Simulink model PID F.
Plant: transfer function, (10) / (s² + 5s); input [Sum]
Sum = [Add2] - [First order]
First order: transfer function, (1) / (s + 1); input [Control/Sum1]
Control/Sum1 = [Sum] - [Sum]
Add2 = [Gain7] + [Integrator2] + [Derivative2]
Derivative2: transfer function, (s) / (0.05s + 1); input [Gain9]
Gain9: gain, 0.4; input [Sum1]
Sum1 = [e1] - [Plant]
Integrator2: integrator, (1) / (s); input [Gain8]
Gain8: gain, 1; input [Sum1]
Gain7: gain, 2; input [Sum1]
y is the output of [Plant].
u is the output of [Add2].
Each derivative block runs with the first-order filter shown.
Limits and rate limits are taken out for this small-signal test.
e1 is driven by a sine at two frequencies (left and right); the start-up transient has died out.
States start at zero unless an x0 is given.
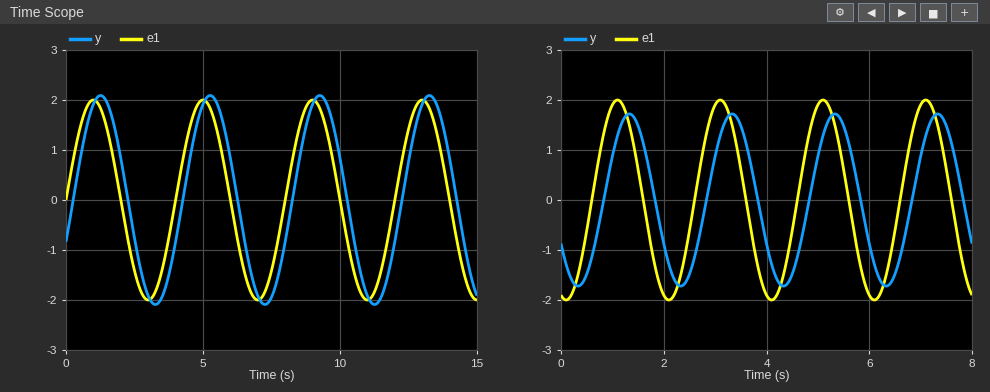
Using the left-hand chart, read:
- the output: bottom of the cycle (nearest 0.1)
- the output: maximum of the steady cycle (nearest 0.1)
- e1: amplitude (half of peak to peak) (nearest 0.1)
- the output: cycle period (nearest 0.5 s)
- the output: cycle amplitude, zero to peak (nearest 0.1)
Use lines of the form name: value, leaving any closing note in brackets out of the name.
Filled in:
the output: bottom of the cycle: -2.1
the output: maximum of the steady cycle: 2.1
e1: amplitude (half of peak to peak): 2.0
the output: cycle period: 4.0 s
the output: cycle amplitude, zero to peak: 2.1
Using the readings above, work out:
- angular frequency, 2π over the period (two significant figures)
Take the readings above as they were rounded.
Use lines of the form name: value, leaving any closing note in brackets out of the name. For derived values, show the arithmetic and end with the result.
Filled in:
angular frequency, 2π over the period: 2π / 4 = 1.6 rad/s
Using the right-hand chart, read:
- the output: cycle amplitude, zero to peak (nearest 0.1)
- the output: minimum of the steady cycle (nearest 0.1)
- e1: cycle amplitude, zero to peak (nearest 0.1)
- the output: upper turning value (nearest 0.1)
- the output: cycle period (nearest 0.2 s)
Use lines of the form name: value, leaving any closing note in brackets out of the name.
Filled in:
the output: cycle amplitude, zero to peak: 1.7
the output: minimum of the steady cycle: -1.7
e1: cycle amplitude, zero to peak: 2.0
the output: upper turning value: 1.7
the output: cycle period: 2.0 s
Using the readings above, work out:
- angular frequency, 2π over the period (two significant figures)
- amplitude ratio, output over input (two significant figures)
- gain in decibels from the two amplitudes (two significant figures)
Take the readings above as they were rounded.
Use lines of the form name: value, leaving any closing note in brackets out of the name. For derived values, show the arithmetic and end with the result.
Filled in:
angular frequency, 2π over the period: 2π / 2 = 3.1 rad/s
amplitude ratio, output over input: 1.7 / 2 = 0.85
gain in decibels from the two amplitudes: 20 log10(1.7 / 2) = -1.4 dB
